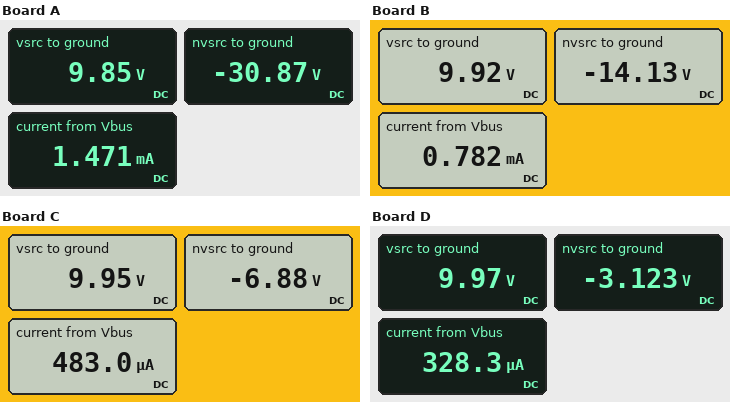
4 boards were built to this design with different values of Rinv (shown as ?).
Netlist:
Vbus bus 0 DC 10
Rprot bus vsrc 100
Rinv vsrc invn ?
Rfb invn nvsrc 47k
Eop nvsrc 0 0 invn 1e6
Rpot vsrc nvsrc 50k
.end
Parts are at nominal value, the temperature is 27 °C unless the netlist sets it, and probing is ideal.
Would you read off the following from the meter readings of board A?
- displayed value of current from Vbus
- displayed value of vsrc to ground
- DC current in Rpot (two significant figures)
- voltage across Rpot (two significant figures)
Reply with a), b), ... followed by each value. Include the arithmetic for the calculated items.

a) 1.471 mA
b) 9.85 V
c) (9.85 V - (-30.87 V)) / 50 kΩ = 810 µA
d) 9.85 V - (-30.87 V) = 41 V
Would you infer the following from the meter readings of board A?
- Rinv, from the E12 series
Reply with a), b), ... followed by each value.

a) 15 kΩ
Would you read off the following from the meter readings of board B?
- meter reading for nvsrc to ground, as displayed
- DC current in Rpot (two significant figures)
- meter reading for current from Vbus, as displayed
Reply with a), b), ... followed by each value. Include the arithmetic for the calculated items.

a) -14.13 V
b) (9.92 V - (-14.13 V)) / 50 kΩ = 480 µA
c) 0.782 mA
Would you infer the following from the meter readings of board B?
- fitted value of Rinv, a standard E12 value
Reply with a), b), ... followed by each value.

a) 33 kΩ
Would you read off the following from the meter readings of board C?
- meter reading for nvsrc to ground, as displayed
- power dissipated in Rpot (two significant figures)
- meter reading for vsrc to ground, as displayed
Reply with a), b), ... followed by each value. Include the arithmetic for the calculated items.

a) -6.88 V
b) (9.95 V - (-6.88 V))^2 / 50 kΩ = 5.7 mW
c) 9.95 V
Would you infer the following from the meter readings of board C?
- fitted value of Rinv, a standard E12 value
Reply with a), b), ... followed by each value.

a) 68 kΩ
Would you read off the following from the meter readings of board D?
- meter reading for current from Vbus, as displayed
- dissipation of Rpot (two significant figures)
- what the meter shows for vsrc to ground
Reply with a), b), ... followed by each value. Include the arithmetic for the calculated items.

a) 328.3 µA
b) (9.97 V - (-3.123 V))^2 / 50 kΩ = 3.4 mW
c) 9.97 V
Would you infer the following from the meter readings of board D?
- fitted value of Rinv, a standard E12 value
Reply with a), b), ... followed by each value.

a) 150 kΩ
